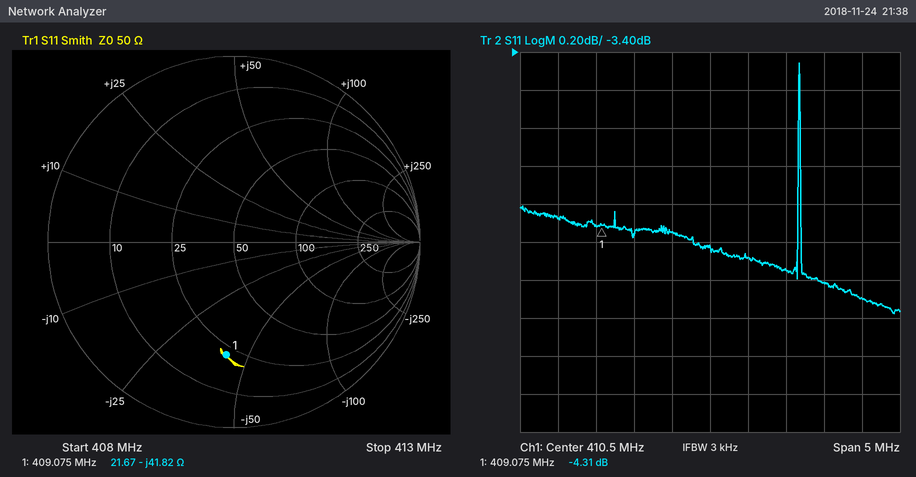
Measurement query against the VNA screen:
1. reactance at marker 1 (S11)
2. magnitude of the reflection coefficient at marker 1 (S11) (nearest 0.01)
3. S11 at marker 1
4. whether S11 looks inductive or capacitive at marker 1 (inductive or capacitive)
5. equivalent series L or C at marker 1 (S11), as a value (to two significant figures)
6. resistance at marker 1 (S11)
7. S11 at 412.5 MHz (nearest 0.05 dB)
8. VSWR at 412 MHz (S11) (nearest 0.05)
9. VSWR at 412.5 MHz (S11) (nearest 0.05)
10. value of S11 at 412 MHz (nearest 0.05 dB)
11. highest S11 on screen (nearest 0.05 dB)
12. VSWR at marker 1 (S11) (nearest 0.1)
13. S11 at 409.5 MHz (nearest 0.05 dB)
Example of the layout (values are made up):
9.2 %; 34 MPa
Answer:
-41.82 Ω; 0.61; -4.31 dB; capacitive; 9.3 pF; 21.67 Ω; -4.70 dB; 3.85; 3.80; -4.60 dB; -3.45 dB; 4.1; -4.35 dB
